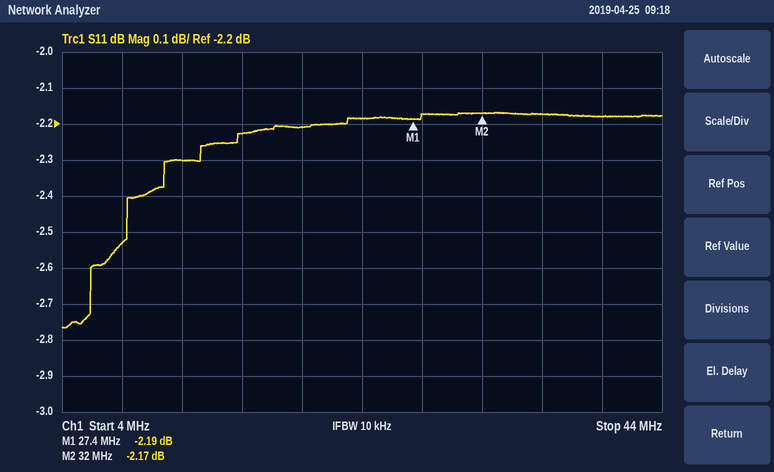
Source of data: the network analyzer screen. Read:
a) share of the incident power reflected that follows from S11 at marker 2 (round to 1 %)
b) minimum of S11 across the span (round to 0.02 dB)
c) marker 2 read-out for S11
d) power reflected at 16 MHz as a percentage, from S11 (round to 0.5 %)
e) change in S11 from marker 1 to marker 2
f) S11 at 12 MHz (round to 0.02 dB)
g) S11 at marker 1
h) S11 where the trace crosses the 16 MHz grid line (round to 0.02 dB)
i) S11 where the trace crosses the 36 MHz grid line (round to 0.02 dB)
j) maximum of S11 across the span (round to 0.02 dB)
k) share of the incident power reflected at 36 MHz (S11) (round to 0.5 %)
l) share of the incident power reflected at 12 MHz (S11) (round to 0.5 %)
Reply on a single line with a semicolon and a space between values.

61 %; -2.76 dB; -2.17 dB; 60.0 %; 0.02 dB; -2.30 dB; -2.19 dB; -2.22 dB; -2.18 dB; -2.16 dB; 60.5 %; 59.0 %
